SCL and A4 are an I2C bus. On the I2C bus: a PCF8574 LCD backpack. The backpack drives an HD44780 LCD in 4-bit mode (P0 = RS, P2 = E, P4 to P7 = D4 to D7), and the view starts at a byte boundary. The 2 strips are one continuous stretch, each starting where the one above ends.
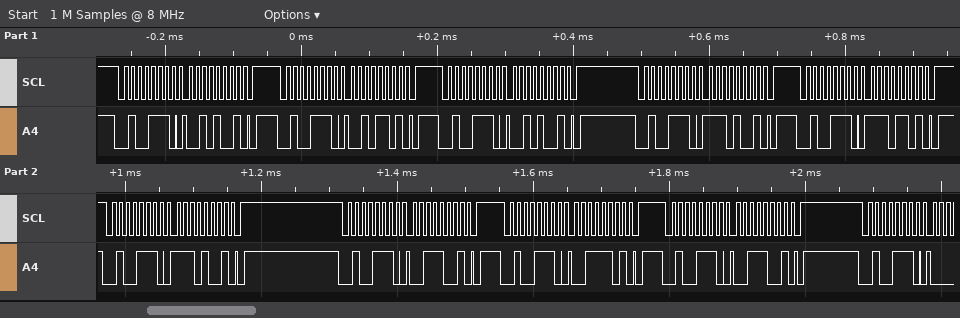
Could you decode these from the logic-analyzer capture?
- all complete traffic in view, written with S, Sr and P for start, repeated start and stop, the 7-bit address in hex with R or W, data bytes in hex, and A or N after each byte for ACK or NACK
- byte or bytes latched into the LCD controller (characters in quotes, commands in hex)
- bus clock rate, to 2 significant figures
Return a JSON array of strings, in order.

["S 27W A 29 A P S 27W A 2D A P S 27W A 29 A P S 27W A E9 A P S 27W A ED A P S 27W A E9 A P S 27W A 39 A P S 27W A 3D A P S 27W A 39 A P S 27W A", "'.'", "100 kHz"]
